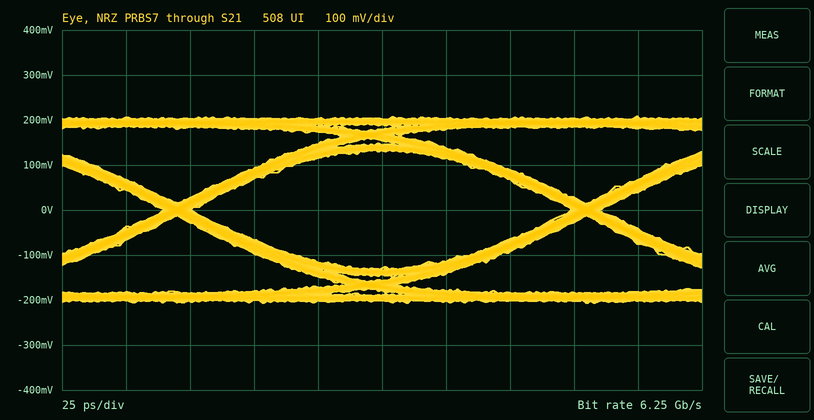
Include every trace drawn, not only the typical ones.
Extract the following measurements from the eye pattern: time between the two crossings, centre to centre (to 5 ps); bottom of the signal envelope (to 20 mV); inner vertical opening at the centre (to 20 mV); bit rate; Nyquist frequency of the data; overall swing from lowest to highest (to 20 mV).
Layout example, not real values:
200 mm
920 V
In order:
160 ps
-200 mV
260 mV
6.25 Gb/s
3.125 GHz
420 mV
